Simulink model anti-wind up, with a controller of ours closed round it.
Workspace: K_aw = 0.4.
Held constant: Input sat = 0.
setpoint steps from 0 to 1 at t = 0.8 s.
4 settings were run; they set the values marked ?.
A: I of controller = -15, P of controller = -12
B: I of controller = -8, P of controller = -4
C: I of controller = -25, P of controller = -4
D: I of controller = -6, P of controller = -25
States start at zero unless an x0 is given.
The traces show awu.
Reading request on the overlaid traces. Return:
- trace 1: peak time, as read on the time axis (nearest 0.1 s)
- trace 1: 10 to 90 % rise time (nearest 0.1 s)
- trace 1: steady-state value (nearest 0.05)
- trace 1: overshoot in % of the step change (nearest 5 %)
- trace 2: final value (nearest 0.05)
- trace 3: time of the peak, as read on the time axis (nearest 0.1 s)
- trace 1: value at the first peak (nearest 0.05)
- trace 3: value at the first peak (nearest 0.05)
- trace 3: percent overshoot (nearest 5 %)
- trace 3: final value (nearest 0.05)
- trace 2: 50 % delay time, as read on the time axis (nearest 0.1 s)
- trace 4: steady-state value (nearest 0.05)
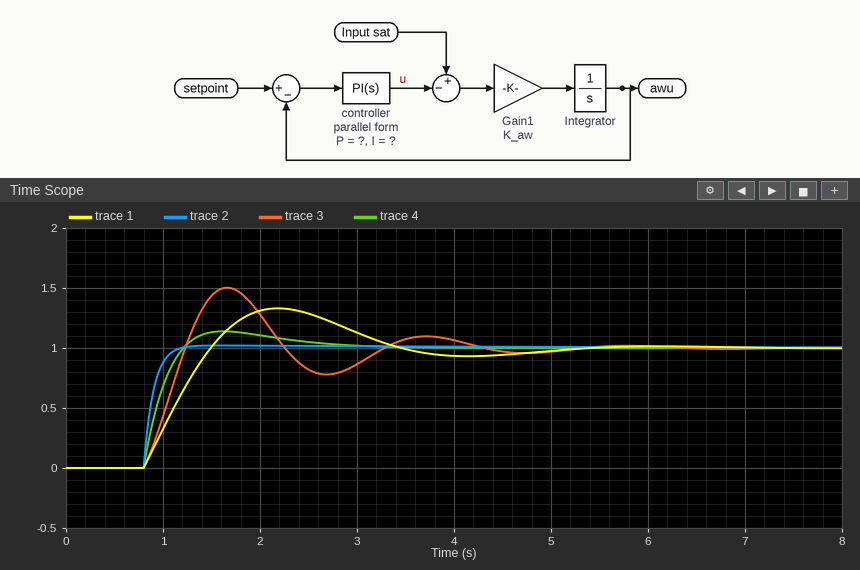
2.2 s
0.5 s
1.00
35 %
1.00
1.7 s
1.35
1.50
50 %
1.00
0.9 s
1.00
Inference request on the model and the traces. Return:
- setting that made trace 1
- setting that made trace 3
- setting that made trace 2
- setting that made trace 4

B
C
D
A
